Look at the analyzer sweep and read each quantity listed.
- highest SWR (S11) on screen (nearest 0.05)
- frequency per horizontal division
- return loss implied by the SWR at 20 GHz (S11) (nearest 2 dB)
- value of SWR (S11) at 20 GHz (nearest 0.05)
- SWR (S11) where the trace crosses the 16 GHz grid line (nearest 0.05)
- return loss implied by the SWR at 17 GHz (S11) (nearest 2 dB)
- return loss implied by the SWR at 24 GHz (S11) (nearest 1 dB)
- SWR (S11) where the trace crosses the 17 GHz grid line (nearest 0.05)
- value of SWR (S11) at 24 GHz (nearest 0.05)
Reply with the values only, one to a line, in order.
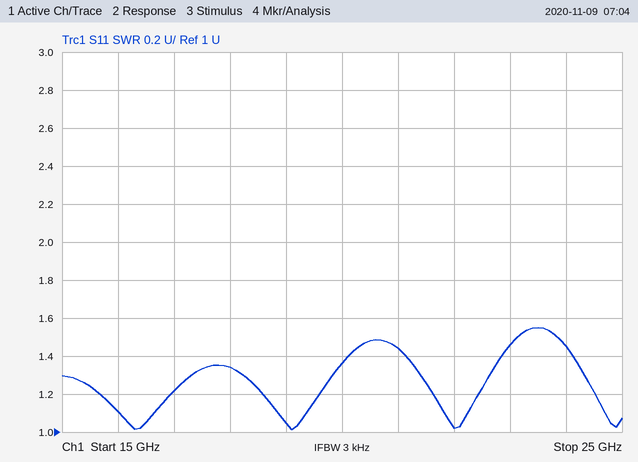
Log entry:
1.55
1 GHz
16 dB
1.35
1.10
20 dB
15 dB
1.20
1.45
